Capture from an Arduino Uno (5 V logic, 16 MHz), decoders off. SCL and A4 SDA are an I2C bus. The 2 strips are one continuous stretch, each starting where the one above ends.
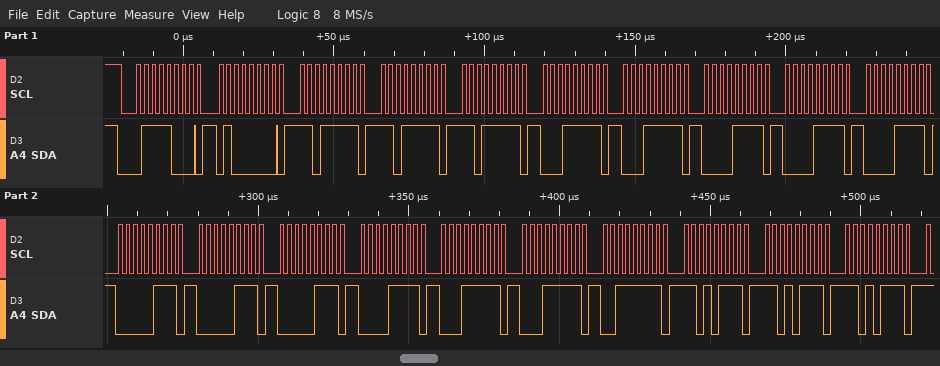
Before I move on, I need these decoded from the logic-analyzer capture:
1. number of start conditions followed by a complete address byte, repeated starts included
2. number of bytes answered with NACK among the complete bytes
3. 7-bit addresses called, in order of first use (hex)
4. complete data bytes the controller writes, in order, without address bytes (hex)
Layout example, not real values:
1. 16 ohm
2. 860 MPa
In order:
1. 1
2. 0
3. 0x3C
4. 40 DF DF DF 1F 1F 0F 0F 0F 07 07 07 0F 1F 1F 3F D7 D7 D7
